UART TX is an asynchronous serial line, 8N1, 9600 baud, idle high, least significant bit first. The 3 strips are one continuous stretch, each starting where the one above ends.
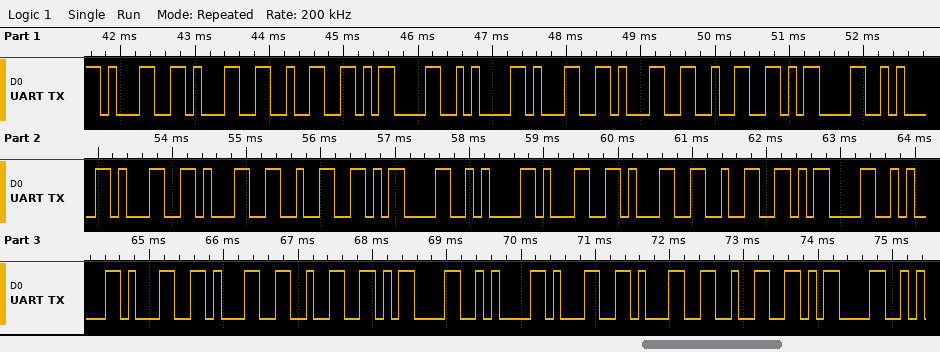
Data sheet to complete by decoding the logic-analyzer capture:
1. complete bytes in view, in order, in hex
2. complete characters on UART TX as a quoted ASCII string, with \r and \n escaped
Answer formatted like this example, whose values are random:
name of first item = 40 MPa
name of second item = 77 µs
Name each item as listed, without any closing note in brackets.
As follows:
complete bytes in view, in order, in hex = 0x31 0x31 0x32 0x0D 0x0A 0x31 0x31 0x32 0x0D 0x0A 0x31 0x31 0x32 0x0D 0x0A 0x31 0x31 0x32 0x0D 0x0A 0x31 0x31 0x32 0x0D 0x0A 0x31 0x31 0x32 0x0D
complete characters on UART TX as a quoted ASCII string, with \r and \n escaped = "112\r\n112\r\n112\r\n112\r\n112\r\n112\r"
